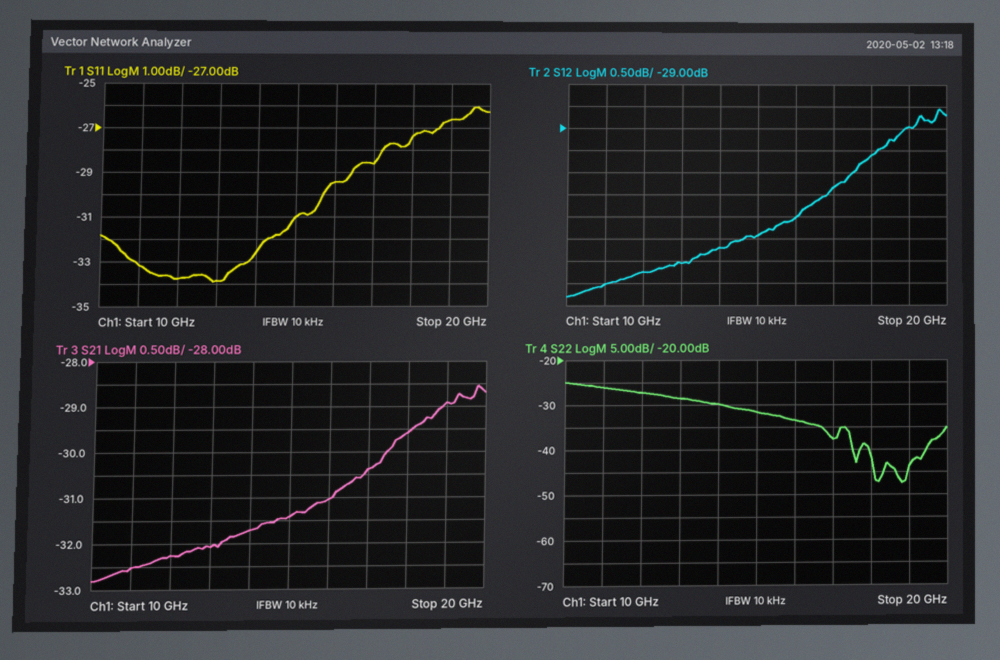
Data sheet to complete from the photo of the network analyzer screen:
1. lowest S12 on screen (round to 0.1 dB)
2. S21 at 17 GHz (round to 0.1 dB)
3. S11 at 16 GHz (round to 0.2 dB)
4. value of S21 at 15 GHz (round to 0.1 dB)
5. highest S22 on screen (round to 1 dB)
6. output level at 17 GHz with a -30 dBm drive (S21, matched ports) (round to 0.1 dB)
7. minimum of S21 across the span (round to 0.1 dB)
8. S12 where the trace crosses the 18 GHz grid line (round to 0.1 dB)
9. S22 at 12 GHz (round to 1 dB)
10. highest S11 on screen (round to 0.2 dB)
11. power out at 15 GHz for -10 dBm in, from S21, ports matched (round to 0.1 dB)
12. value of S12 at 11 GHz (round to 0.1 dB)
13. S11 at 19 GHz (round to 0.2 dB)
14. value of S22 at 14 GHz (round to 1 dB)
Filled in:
-32.8 dB
-30.4 dB
-29.4 dB
-31.4 dB
-25 dB
-60.4 dBm
-32.8 dB
-29.6 dB
-27 dB
-26.0 dB
-41.4 dBm
-32.5 dB
-26.6 dB
-30 dB
